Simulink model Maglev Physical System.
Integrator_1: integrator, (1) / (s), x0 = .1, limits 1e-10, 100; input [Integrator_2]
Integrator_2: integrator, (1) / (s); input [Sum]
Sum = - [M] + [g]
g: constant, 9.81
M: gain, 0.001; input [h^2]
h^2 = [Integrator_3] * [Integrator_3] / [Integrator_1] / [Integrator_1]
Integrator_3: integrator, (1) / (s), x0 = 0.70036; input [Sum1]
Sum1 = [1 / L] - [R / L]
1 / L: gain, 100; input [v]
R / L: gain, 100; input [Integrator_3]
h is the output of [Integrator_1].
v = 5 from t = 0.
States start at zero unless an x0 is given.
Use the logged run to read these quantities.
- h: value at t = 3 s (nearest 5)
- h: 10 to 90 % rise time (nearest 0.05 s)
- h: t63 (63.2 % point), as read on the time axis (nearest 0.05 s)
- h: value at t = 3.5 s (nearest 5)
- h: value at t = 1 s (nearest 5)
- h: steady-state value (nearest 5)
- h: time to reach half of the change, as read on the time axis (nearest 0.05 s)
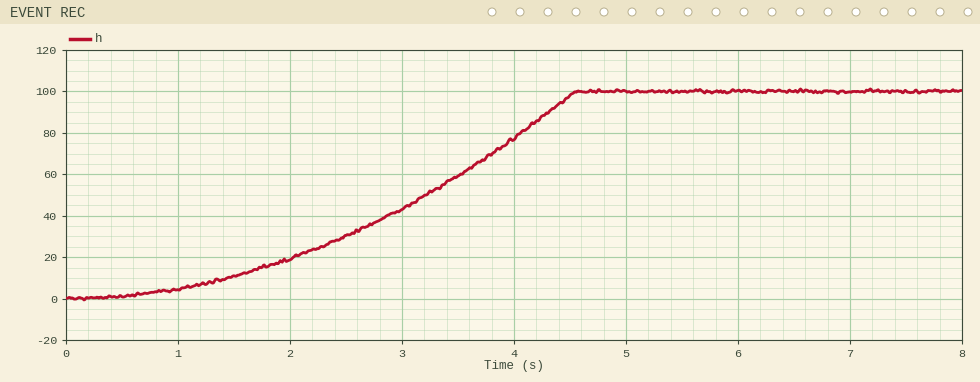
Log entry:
45
2.85 s
3.60 s
60
5
100
3.20 s
